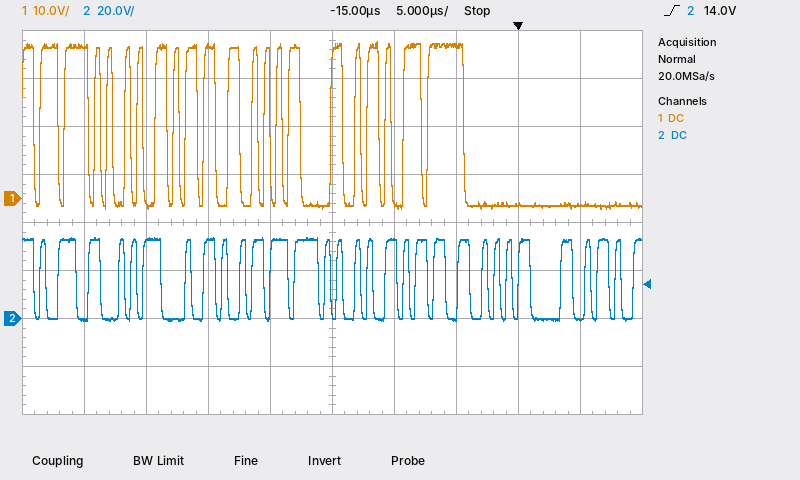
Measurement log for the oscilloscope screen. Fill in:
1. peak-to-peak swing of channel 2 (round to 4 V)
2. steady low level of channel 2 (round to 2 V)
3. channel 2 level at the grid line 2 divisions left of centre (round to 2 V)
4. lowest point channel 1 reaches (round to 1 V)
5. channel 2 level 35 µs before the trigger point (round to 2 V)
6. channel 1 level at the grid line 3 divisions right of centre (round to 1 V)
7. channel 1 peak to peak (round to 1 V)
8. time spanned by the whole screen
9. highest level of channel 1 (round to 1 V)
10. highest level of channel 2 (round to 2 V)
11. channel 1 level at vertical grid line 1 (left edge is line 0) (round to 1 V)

36 V
0 V
32 V
-2 V
0 V
-1 V
35 V
50 µs
33 V
34 V
32 V
